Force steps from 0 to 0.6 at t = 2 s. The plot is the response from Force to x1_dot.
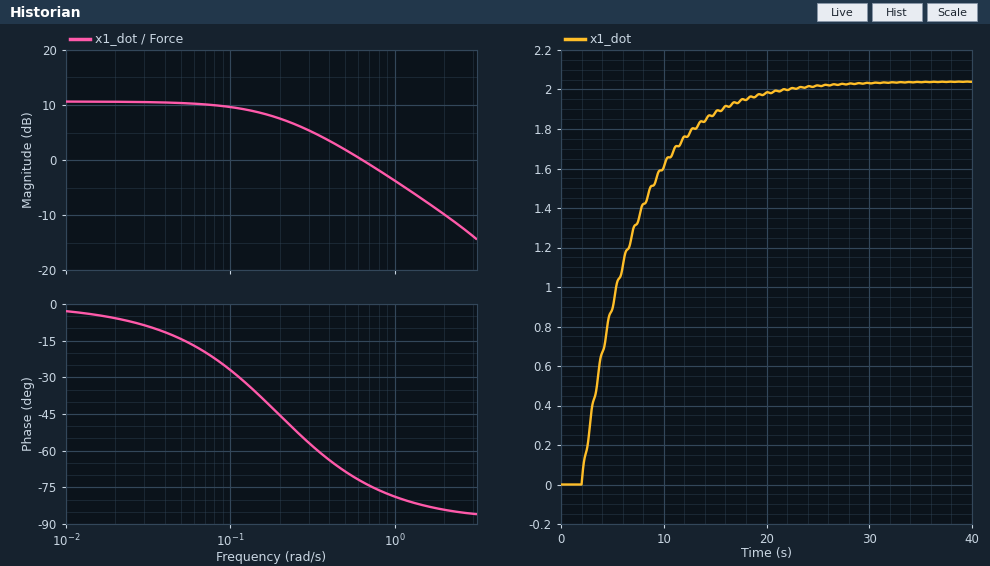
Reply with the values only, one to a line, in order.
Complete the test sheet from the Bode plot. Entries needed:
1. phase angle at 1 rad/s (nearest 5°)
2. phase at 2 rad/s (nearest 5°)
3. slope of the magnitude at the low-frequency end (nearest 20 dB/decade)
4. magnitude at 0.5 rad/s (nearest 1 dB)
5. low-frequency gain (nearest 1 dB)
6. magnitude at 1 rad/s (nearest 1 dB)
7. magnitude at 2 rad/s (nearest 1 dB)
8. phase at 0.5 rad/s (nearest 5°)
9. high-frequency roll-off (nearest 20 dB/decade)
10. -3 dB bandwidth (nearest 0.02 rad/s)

-80°
-85°
0 dB/decade
2 dB
11 dB
-4 dB
-10 dB
-70°
-20 dB/decade
0.20 rad/s
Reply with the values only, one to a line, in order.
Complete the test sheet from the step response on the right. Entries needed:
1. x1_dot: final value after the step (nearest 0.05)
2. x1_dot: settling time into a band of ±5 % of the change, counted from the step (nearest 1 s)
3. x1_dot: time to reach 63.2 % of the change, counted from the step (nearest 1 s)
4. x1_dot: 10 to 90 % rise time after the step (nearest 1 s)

2.05
15 s
5 s
11 s
